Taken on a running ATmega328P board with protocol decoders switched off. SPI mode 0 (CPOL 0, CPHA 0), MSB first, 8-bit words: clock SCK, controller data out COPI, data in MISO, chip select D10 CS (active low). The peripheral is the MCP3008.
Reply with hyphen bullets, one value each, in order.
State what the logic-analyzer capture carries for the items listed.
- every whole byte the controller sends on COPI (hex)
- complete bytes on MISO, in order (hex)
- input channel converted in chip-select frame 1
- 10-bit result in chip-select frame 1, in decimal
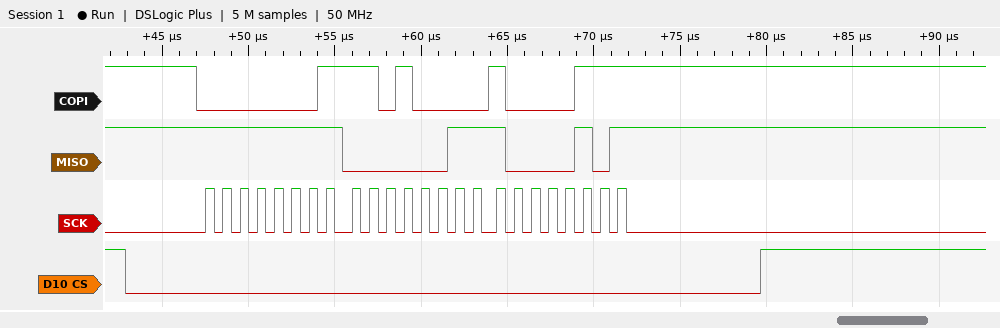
- 0x01 0xD0 0x87
- 0xFF 0x03 0x85
- 5
- 901
